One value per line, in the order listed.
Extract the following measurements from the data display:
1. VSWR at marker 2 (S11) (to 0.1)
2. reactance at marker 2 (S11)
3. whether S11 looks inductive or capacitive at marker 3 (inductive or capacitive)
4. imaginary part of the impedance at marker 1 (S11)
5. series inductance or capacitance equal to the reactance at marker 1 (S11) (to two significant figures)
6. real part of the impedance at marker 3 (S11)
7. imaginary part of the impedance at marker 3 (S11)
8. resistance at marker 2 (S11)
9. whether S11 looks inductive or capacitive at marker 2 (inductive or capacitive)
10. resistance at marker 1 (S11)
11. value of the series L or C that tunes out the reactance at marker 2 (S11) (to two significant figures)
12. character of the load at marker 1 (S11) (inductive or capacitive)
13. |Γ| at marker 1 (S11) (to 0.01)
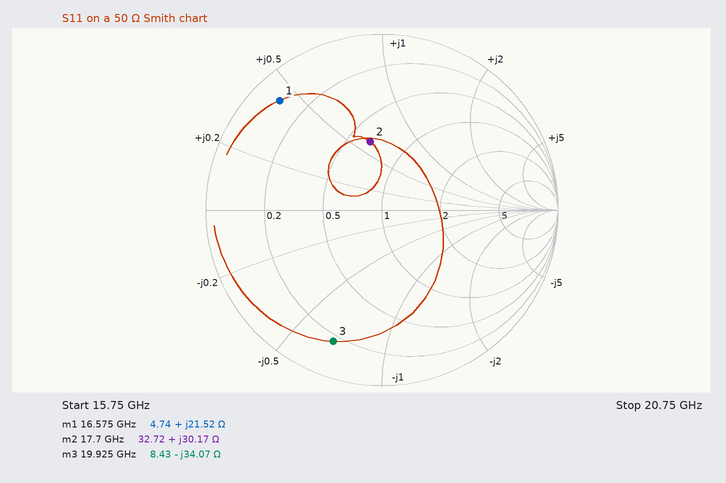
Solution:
2.3
+30.17 Ω
capacitive
+21.52 Ω
210 pH
8.43 Ω
-34.07 Ω
32.72 Ω
inductive
4.74 Ω
300 fF
inductive
0.85
